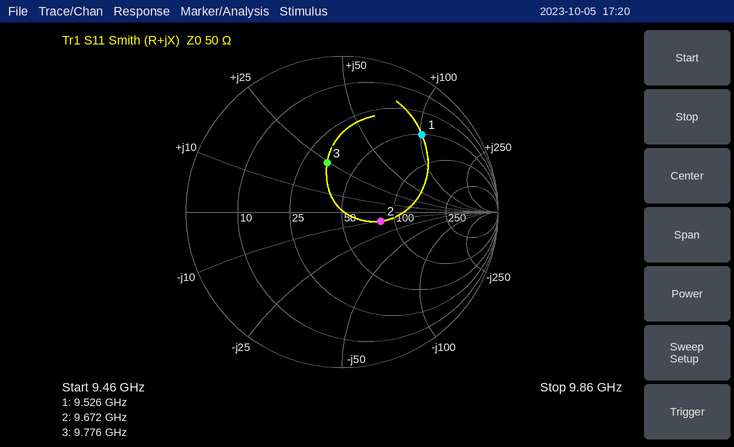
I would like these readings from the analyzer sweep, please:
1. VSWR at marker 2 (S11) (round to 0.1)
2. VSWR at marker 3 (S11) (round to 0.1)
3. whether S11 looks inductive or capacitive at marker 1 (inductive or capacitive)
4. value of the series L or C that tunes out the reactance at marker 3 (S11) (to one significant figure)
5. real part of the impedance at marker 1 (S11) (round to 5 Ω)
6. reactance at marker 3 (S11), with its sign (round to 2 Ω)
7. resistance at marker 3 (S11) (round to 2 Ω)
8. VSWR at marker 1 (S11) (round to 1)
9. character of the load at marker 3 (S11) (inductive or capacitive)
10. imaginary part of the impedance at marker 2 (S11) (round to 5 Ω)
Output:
1.7
2.0
inductive
700 fF
50 Ω
+24 Ω
34 Ω
6
inductive
-10 Ω
